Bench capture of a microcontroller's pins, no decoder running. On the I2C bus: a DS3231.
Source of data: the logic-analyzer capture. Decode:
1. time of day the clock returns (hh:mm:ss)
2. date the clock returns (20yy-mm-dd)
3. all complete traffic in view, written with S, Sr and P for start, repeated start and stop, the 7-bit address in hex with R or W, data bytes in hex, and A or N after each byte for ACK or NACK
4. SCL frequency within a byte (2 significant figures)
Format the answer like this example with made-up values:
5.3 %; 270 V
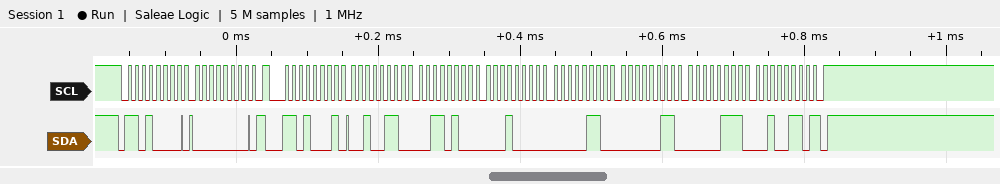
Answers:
10:34:26; 2026-07-03; S 68W A 00 A Sr 68R A 26 A 34 A 10 A 06 A 03 A 07 A 26 N P; 100 kHz
